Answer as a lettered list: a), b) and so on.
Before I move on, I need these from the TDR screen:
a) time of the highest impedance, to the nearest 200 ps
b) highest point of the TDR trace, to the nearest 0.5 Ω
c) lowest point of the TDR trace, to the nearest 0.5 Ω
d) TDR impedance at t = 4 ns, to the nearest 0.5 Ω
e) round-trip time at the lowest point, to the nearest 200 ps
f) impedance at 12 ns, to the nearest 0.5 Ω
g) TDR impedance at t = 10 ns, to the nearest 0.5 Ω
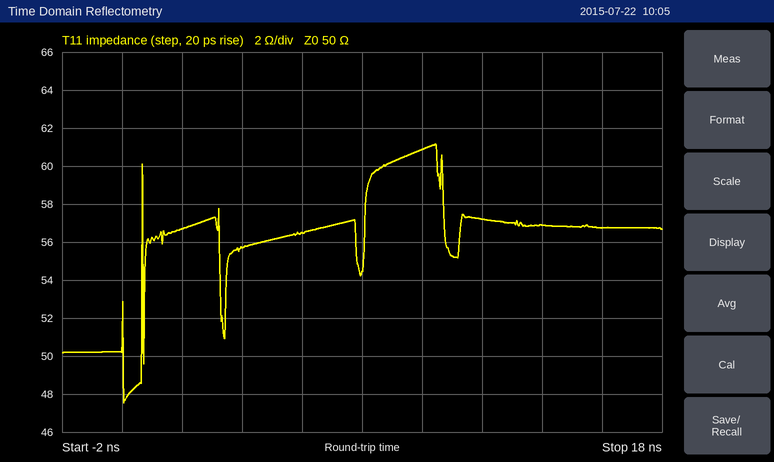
a) 10.4 ns
b) 61.0 Ω
c) 47.5 Ω
d) 55.5 Ω
e) 0.0 ns
f) 57.0 Ω
g) 61.0 Ω
